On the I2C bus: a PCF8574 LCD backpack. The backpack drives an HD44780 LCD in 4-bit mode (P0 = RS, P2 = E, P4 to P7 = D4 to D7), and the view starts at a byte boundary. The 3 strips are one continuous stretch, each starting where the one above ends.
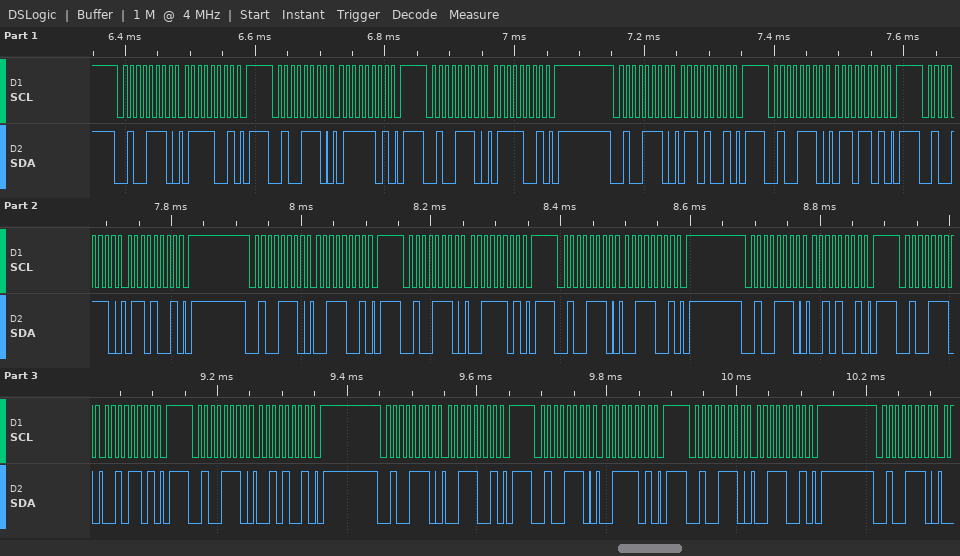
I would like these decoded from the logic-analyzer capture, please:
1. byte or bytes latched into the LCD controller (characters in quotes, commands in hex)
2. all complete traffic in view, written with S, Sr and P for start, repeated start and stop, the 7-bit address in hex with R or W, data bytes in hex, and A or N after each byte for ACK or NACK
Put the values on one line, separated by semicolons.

'v' '2'; S 27W A 79 A P S 27W A 7D A P S 27W A 79 A P S 27W A 69 A P S 27W A 6D A P S 27W A 69 A P S 27W A 39 A P S 27W A 3D A P S 27W A 39 A P S 27W A 29 A P S 27W A 2D A P S 27W A 29 A P S 27W A 39 A P S 27W A 3D A P S 27W A 39 A P S 27W A
